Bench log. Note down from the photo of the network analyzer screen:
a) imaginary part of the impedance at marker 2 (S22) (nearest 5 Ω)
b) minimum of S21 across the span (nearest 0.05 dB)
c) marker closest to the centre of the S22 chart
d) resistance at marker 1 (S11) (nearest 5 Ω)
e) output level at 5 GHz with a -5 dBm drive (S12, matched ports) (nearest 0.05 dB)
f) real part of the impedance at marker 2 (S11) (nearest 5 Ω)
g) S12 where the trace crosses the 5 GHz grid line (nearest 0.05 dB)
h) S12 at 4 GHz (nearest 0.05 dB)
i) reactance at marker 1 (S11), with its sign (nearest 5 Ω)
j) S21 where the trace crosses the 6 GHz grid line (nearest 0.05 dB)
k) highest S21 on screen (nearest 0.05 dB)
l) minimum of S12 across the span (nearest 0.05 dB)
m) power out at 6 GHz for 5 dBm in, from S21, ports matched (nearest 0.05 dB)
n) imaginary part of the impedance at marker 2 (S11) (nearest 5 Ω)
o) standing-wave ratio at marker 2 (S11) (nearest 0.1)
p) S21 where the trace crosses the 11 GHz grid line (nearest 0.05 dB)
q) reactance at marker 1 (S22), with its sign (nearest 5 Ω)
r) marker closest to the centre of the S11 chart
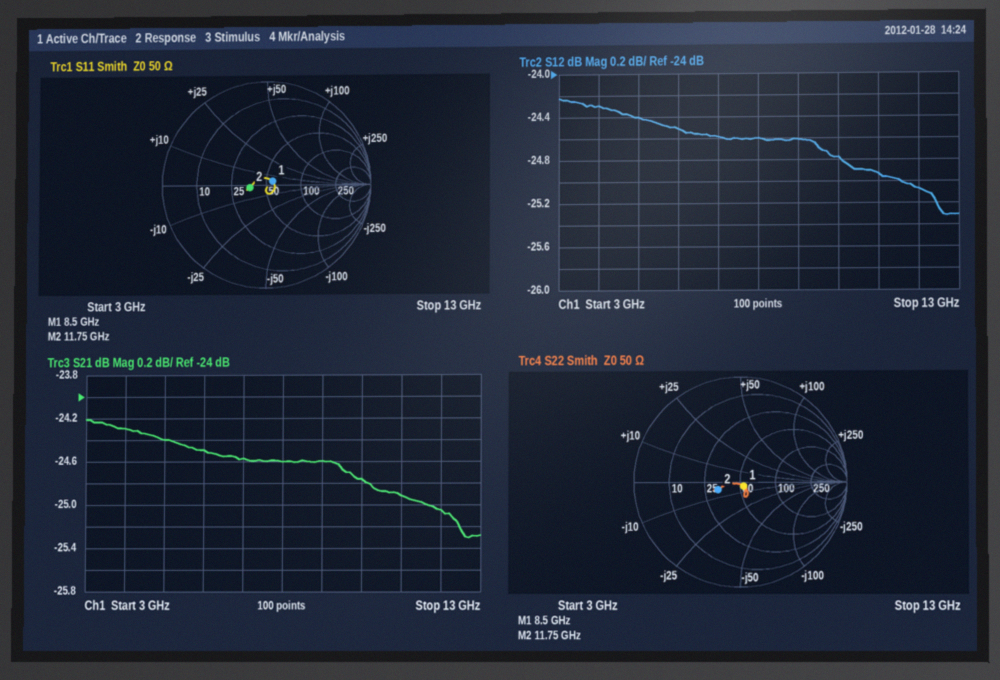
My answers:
-5 Ω
-25.30 dB
marker 1
55 Ω
-29.40 dBm
35 Ω
-24.40 dB
-24.30 dB
+5 Ω
-24.50 dB
-24.20 dB
-25.30 dB
-19.50 dBm
0 Ω
1.4
-24.90 dB
-5 Ω
marker 1
